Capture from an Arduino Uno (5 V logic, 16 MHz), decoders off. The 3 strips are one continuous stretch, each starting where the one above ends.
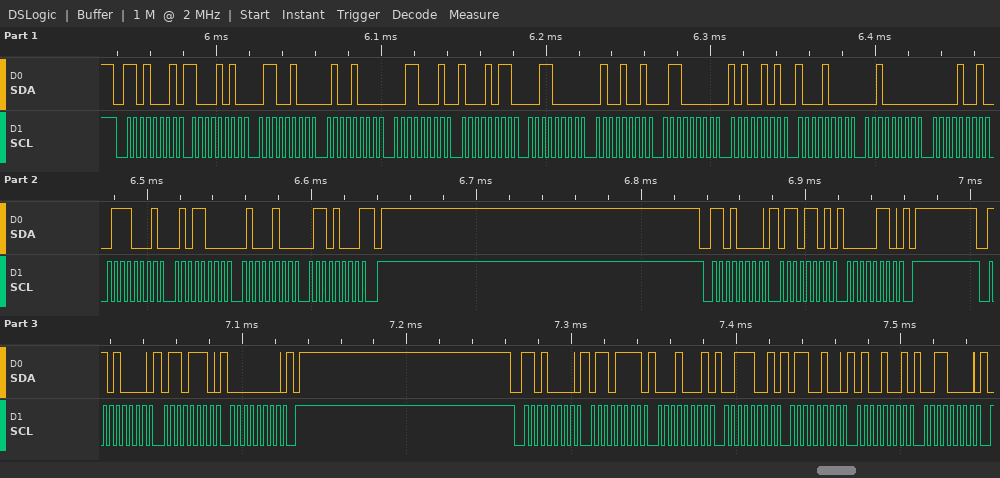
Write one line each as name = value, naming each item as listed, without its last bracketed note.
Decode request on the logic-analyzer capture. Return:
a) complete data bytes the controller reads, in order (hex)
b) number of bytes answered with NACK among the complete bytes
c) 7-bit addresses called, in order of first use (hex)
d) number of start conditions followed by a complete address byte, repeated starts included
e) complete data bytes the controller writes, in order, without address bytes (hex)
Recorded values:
complete data bytes the controller reads, in order = 8A 64 48 31 8B 30 49 60 A5 88 20 09 71 58 44 68
number of bytes answered with NACK among the complete bytes = 1
7-bit addresses called, in order of first use = 0x68
number of start conditions followed by a complete address byte, repeated starts included = 4
complete data bytes the controller writes, in order, without address bytes = 6D 06 6E 00 6F 11 39 64 49 30
